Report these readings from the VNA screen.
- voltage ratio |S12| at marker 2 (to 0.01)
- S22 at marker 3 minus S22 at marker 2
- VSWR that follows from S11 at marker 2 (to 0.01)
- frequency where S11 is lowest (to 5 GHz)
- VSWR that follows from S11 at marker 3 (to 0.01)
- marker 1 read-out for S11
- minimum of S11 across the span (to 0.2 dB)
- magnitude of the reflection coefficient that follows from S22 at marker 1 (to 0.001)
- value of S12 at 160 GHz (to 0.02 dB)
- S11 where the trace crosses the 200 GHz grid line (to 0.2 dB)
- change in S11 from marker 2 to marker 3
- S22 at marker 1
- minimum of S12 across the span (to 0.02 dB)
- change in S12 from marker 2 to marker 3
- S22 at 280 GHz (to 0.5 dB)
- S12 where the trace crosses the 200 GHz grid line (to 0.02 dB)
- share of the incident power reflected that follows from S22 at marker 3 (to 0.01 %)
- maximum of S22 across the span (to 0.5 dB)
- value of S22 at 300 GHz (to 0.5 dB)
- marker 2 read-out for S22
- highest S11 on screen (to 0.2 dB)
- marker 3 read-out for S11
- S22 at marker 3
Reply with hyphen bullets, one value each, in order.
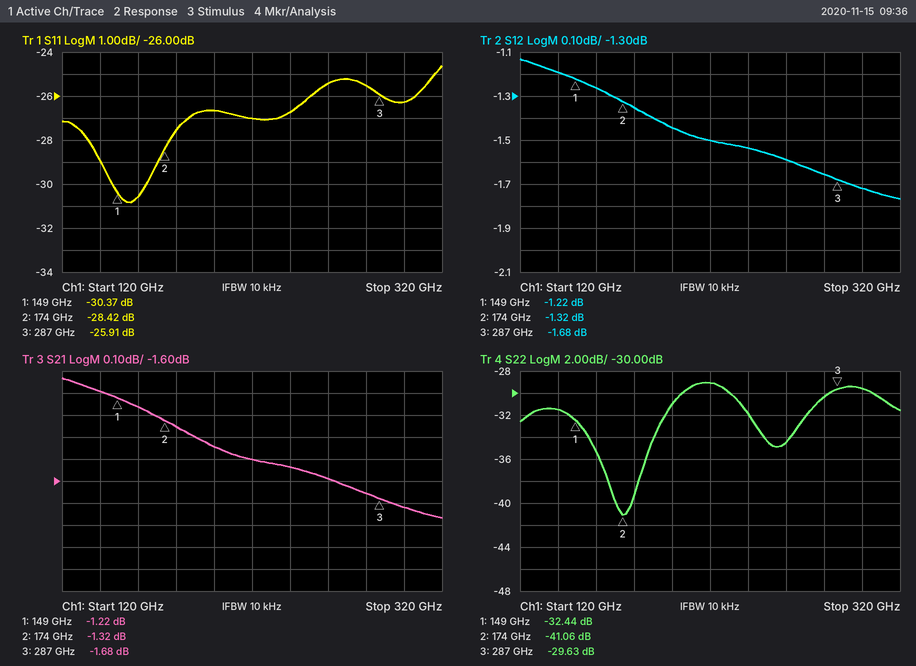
- 0.86
- 11.43 dB
- 1.08
- 155 GHz
- 1.11
- -30.37 dB
- -30.8 dB
- 0.024
- -1.26 dB
- -26.6 dB
- 2.51 dB
- -32.44 dB
- -1.76 dB
- -0.36 dB
- -30.5 dB
- -1.44 dB
- 0.11 %
- -29.0 dB
- -29.5 dB
- -41.06 dB
- -24.6 dB
- -25.91 dB
- -29.63 dB
